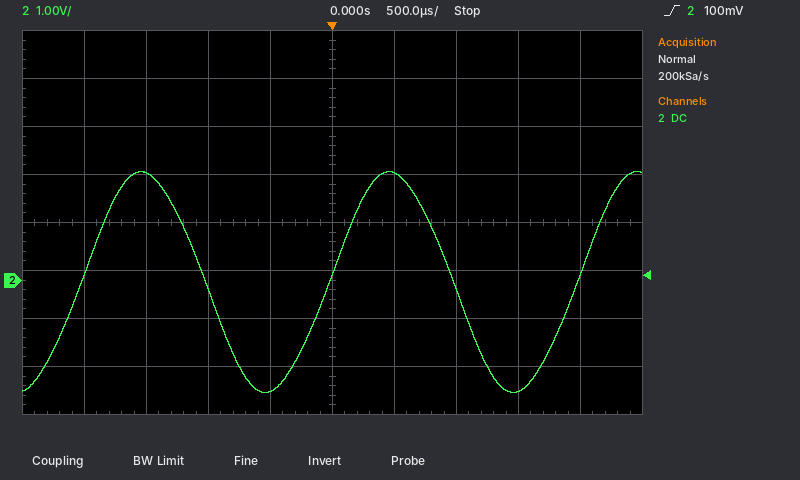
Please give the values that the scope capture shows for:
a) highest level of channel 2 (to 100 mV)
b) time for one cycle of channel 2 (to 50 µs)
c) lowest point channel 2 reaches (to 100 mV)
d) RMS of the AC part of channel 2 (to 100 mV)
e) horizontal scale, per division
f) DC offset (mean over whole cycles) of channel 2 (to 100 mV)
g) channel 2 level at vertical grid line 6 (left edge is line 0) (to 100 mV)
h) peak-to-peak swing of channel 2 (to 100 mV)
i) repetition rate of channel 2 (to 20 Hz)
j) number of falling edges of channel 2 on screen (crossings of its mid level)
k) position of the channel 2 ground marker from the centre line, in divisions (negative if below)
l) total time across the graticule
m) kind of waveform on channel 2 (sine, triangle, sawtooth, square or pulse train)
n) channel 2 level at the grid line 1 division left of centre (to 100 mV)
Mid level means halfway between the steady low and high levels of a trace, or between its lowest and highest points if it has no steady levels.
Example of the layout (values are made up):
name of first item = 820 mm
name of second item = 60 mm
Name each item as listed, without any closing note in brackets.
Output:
highest level of channel 2 = 2.3 V
time for one cycle of channel 2 = 2.00 ms
lowest point channel 2 reaches = -2.3 V
RMS of the AC part of channel 2 = 1.6 V
horizontal scale, per division = 500 µs
DC offset (mean over whole cycles) of channel 2 = 0.0 V
channel 2 level at vertical grid line 6 (left edge is line 0) = 2.2 V
peak-to-peak swing of channel 2 = 4.6 V
repetition rate of channel 2 = 500 Hz
number of falling edges of channel 2 on screen = 2
position of the channel 2 ground marker from the centre line, in divisions = -1.2 div
total time across the graticule = 5 ms
kind of waveform on channel 2 = sine
channel 2 level at the grid line 1 division left of centre = -2.3 V
